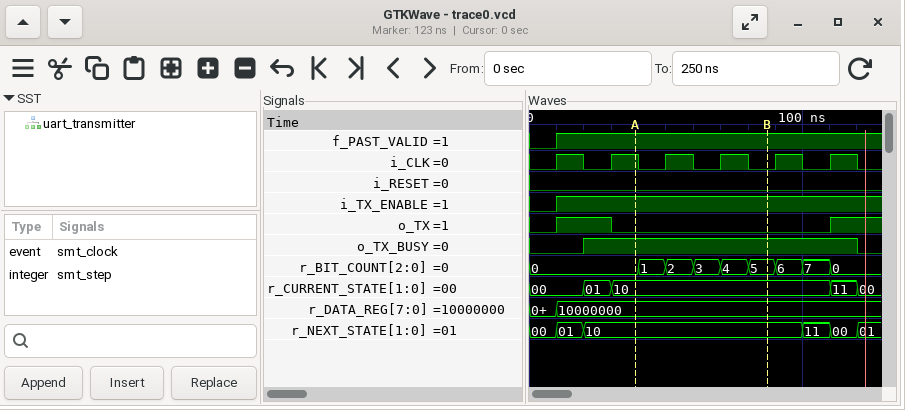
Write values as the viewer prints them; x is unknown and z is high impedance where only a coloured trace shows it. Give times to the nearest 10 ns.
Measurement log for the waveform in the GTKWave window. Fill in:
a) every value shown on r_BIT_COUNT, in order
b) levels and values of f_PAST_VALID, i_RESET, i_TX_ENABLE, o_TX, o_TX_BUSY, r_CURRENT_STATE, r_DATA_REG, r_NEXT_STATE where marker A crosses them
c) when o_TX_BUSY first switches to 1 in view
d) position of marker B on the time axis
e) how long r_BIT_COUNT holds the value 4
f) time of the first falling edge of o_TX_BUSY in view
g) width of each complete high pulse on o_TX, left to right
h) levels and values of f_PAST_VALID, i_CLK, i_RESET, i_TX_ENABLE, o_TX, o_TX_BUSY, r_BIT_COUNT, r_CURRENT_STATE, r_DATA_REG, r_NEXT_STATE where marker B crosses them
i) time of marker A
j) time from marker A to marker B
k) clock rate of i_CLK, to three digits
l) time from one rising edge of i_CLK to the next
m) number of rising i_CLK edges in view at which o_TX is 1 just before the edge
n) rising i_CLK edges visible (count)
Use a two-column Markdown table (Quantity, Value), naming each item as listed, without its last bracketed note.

| Quantity | Value |
|---|---|
| every value shown on r_BIT_COUNT, in order | 0, 1, 2, 3, 4, 5, 6, 7, 0 |
| levels and values of f_PAST_VALID, i_RESET, i_TX_ENABLE, o_TX, o_TX_BUSY, r_CURRENT_STATE, r_DATA_REG, r_NEXT_STATE where marker A crosses them | f_PAST_VALID=1, i_RESET=0, i_TX_ENABLE=1, o_TX=0, o_TX_BUSY=1, r_CURRENT_STATE=10, r_DATA_REG=10000000, r_NEXT_STATE=10 |
| when o_TX_BUSY first switches to 1 in view | 20 ns |
| position of marker B on the time axis | 90 ns |
| how long r_BIT_COUNT holds the value 4 | 10 ns |
| time of the first falling edge of o_TX_BUSY in view | 120 ns |
| width of each complete high pulse on o_TX, left to right | 20 ns |
| levels and values of f_PAST_VALID, i_CLK, i_RESET, i_TX_ENABLE, o_TX, o_TX_BUSY, r_BIT_COUNT, r_CURRENT_STATE, r_DATA_REG, r_NEXT_STATE where marker B crosses them | f_PAST_VALID=1, i_CLK=0, i_RESET=0, i_TX_ENABLE=1, o_TX=0, o_TX_BUSY=1, r_BIT_COUNT=5, r_CURRENT_STATE=10, r_DATA_REG=10000000, r_NEXT_STATE=10 |
| time of marker A | 40 ns |
| time from marker A to marker B | 50 ns |
| clock rate of i_CLK, to three digits | 50.0 MHz |
| time from one rising edge of i_CLK to the next | 20 ns |
| number of rising i_CLK edges in view at which o_TX is 1 just before the edge | 1 |
| rising i_CLK edges visible | 6 |
